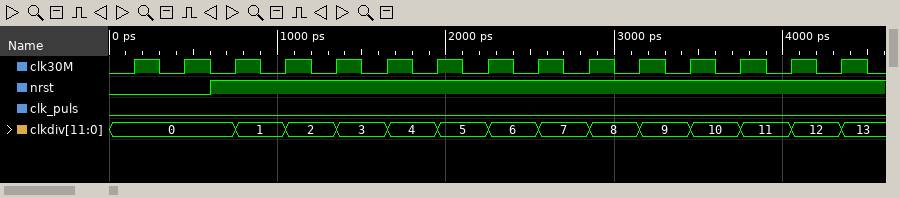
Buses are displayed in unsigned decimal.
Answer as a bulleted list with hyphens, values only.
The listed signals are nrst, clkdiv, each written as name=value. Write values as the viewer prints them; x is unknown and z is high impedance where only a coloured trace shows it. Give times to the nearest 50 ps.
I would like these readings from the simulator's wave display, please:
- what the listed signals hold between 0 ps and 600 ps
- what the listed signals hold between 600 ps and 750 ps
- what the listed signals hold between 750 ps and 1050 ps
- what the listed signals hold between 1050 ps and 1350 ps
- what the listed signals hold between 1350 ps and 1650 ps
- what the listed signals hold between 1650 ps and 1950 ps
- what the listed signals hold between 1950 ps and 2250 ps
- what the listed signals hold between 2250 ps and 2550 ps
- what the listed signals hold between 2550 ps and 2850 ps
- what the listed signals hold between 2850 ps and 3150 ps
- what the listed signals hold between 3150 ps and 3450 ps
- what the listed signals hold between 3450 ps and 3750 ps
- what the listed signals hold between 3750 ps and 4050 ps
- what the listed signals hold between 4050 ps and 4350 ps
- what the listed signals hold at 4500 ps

- nrst=0, clkdiv=0
- nrst=1, clkdiv=0
- nrst=1, clkdiv=1
- nrst=1, clkdiv=2
- nrst=1, clkdiv=3
- nrst=1, clkdiv=4
- nrst=1, clkdiv=5
- nrst=1, clkdiv=6
- nrst=1, clkdiv=7
- nrst=1, clkdiv=8
- nrst=1, clkdiv=9
- nrst=1, clkdiv=10
- nrst=1, clkdiv=11
- nrst=1, clkdiv=12
- nrst=1, clkdiv=13
